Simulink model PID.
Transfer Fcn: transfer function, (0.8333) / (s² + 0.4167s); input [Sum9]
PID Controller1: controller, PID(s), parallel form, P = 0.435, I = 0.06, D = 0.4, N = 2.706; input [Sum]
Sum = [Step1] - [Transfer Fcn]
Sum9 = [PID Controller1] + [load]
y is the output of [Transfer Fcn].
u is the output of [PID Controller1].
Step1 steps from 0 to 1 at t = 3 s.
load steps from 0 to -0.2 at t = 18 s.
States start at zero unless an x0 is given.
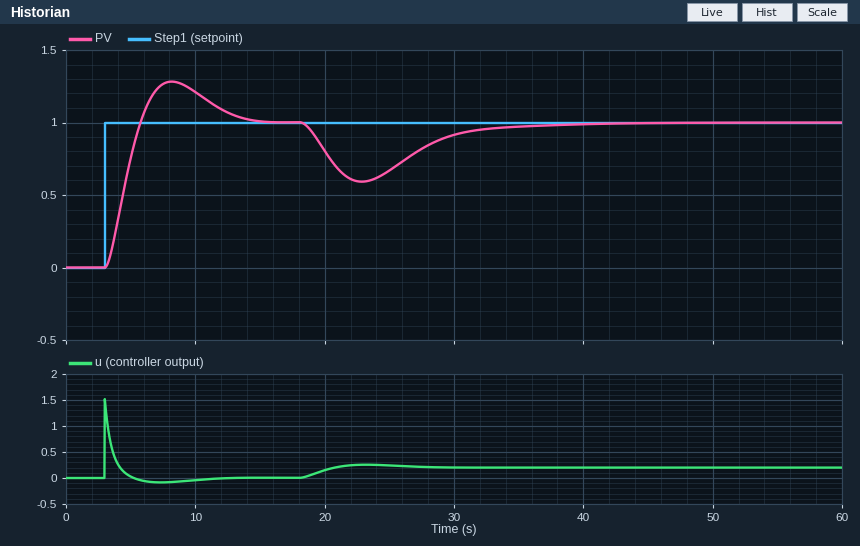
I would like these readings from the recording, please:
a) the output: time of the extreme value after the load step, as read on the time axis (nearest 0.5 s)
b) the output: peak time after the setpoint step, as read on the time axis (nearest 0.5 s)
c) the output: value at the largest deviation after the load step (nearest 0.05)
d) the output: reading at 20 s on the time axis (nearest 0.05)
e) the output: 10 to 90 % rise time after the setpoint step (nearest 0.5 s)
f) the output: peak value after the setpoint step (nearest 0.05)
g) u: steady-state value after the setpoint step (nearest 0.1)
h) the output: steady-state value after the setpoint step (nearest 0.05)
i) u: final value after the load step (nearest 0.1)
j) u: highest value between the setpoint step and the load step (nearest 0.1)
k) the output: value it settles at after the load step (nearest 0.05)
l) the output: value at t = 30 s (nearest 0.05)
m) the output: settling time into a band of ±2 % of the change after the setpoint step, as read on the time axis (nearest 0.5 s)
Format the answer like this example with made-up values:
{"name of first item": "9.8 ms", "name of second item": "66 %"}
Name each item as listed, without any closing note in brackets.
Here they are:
{"the output: time of the extreme value after the load step, as read on the time axis": "23.0 s", "the output: peak time after the setpoint step, as read on the time axis": "8.0 s", "the output: value at the largest deviation after the load step": "0.60", "the output: reading at 20 s on the time axis": "0.80", "the output: 10 to 90 % rise time after the setpoint step": "2.0 s", "the output: peak value after the setpoint step": "1.30", "u: steady-state value after the setpoint step": "0.0", "the output: steady-state value after the setpoint step": "1.00", "u: final value after the load step": "0.2", "u: highest value between the setpoint step and the load step": "1.5", "the output: value it settles at after the load step": "1.00", "the output: value at t = 30 s": "0.90", "the output: settling time into a band of ±2 % of the change after the setpoint step, as read on the time axis": "14.0 s"}
